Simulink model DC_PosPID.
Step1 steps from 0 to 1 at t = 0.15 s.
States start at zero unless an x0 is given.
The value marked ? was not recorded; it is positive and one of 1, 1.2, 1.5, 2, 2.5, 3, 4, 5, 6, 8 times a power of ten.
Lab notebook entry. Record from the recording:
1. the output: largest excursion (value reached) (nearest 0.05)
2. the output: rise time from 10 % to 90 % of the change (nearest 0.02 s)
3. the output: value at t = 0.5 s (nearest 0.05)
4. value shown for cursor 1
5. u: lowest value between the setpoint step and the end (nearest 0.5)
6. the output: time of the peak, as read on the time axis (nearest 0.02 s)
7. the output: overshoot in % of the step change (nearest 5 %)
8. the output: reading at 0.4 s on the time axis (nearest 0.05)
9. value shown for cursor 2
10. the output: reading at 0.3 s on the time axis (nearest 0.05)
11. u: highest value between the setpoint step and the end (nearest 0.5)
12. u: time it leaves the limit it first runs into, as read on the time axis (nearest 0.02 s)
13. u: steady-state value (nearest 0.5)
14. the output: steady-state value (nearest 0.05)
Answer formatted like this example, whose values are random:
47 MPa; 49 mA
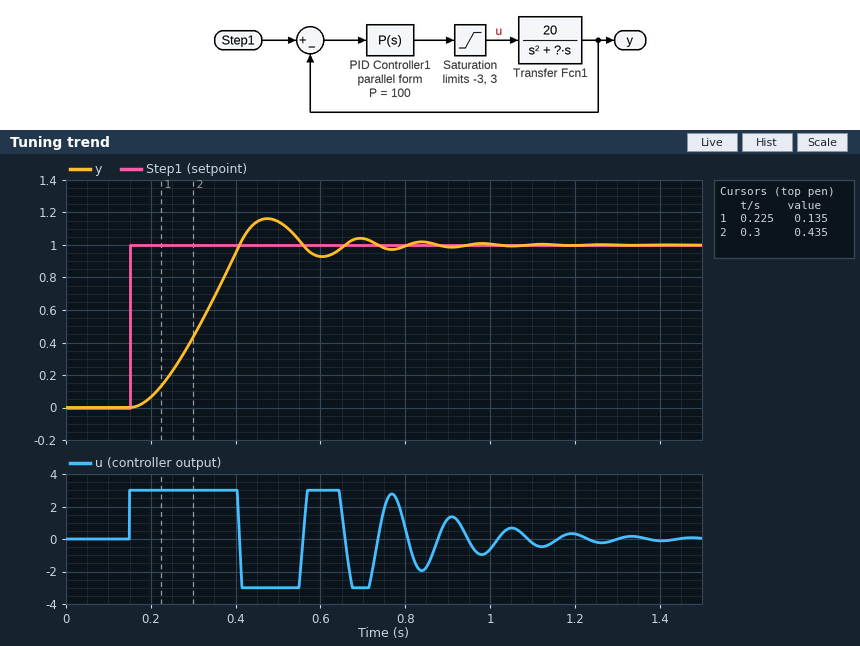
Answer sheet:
1.15; 0.18 s; 1.15; 0.135; -3.0; 0.48 s; 15 %; 0.95; 0.435; 0.45; 3.0; 0.40 s; 0.0; 1.00
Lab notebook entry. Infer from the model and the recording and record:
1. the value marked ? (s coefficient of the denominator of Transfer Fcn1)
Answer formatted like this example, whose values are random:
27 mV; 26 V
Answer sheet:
10
